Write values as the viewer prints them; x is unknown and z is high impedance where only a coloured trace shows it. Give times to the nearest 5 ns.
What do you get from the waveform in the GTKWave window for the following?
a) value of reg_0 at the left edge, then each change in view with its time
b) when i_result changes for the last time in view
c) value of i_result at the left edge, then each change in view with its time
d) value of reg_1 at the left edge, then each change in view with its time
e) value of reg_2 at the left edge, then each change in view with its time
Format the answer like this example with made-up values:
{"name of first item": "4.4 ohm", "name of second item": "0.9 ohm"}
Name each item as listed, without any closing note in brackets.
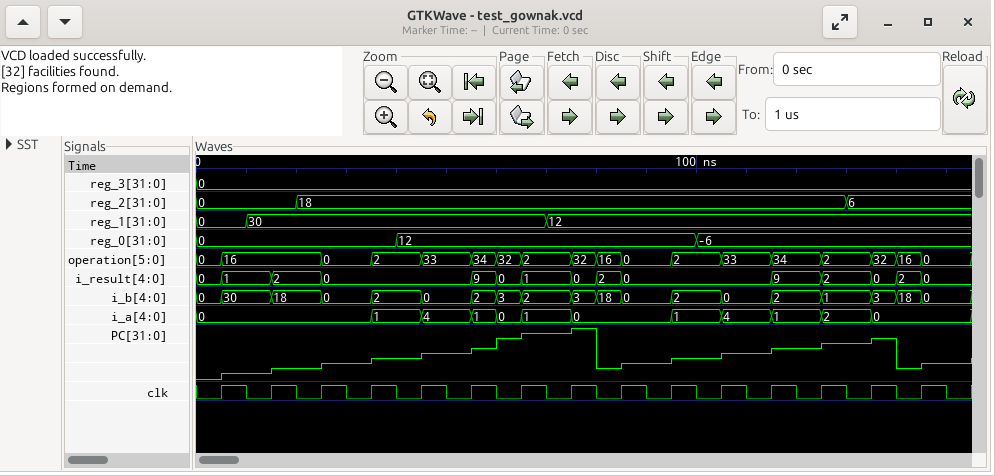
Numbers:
{"value of reg_0 at the left edge, then each change in view with its time": "0, 12 at 40 ns, -6 at 100 ns", "when i_result changes for the last time in view": "145 ns", "value of i_result at the left edge, then each change in view with its time": "0, 1 at 5 ns, 2 at 15 ns, 0 at 25 ns, 9 at 55 ns, 0 at 60 ns, 1 at 65 ns, 0 at 75 ns, 2 at 80 ns, 0 at 85 ns, 9 at 115 ns, 2 at 125 ns, 0 at 135 ns, 2 at 140 ns, 0 at 145 ns", "value of reg_1 at the left edge, then each change in view with its time": "0, 30 at 10 ns, 12 at 70 ns", "value of reg_2 at the left edge, then each change in view with its time": "0, 18 at 20 ns, 6 at 130 ns"}
